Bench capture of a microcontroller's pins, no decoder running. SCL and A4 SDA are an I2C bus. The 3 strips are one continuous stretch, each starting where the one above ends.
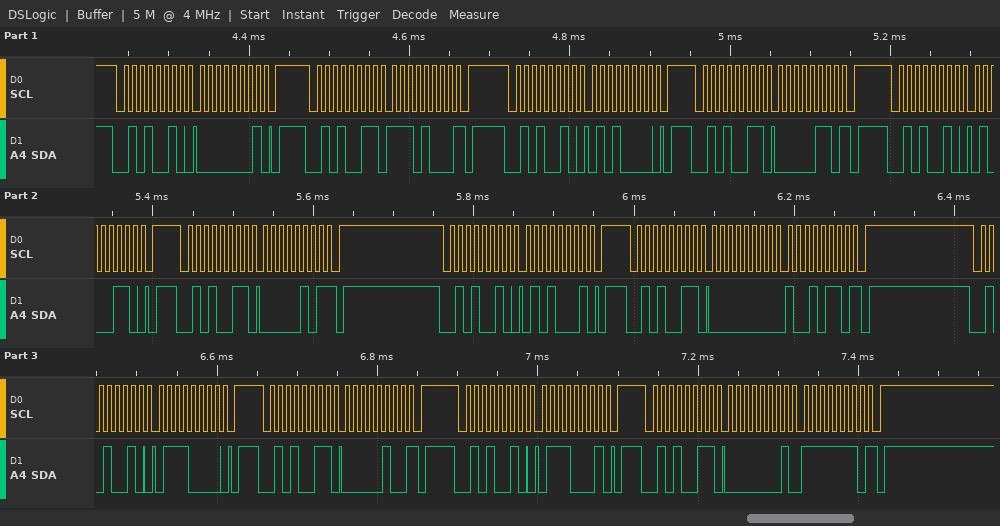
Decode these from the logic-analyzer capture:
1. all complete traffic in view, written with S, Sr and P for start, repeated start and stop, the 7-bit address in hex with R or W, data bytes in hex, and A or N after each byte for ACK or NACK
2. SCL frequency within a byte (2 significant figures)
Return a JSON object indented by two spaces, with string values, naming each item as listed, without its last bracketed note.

{
  "all complete traffic in view, written with S, Sr and P for start, repeated start and stop, the 7-bit address in hex with R or W, data bytes in hex, and A or N after each byte for ACK or NACK": "S 29W A 01 A P S 29R A E8 N P S 29W A 50 A P S 29R A 06 N P S 29W A 46 A P S 29R A 05 N P S 29W A 51 A P S 29R A 00 A 96 N P S 29W A 70 A P S 29R A 04 N P S 29W A 71 A P S 29R A 01 A FE N P",
  "SCL frequency within a byte": "100 kHz"
}
